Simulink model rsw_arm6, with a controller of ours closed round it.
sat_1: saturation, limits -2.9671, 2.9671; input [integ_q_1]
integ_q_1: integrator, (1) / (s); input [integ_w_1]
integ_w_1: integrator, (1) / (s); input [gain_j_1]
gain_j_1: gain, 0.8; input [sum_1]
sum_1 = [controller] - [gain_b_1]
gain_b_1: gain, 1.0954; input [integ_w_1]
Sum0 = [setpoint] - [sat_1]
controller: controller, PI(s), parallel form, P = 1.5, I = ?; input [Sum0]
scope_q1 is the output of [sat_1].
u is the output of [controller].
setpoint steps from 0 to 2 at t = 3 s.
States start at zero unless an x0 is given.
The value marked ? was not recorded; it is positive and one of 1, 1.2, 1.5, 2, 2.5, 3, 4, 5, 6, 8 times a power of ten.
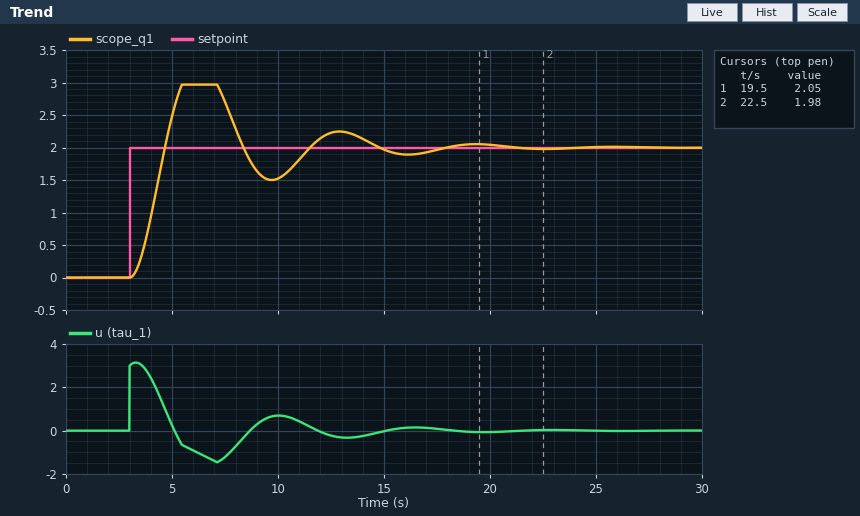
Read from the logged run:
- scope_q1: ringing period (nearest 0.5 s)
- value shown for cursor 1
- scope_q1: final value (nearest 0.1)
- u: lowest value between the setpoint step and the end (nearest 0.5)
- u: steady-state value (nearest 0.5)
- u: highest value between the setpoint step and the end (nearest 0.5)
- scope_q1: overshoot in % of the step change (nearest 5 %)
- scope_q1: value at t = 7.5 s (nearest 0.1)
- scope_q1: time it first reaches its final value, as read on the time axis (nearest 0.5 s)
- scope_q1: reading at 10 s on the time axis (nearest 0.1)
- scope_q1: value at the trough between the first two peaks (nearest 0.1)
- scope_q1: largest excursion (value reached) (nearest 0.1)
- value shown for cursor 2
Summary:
6.5 s
2.05
2.0
-1.5
0.0
3.0
50 %
2.7
4.5 s
1.5
1.5
3.0
1.98
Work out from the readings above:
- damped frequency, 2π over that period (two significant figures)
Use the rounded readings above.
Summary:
0.97 rad/s
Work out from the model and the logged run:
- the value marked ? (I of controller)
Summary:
0.5
